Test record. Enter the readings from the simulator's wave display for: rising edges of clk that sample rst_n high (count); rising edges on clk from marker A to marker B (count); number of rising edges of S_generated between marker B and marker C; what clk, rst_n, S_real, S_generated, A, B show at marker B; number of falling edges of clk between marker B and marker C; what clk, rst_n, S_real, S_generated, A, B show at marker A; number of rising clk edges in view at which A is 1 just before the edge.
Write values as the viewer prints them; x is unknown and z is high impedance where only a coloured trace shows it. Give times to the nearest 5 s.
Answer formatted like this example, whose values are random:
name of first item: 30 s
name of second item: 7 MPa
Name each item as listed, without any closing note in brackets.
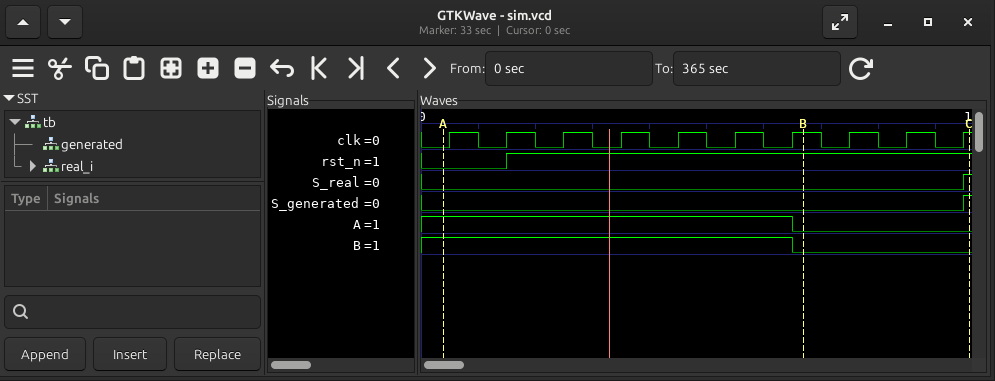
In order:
rising edges of clk that sample rst_n high: 8
rising edges on clk from marker A to marker B: 7
number of rising edges of S_generated between marker B and marker C: 1
what clk, rst_n, S_real, S_generated, A, B show at marker B: clk=1, rst_n=1, S_real=0, S_generated=0, A=0, B=0
number of falling edges of clk between marker B and marker C: 3
what clk, rst_n, S_real, S_generated, A, B show at marker A: clk=0, rst_n=0, S_real=0, S_generated=0, A=1, B=1
number of rising clk edges in view at which A is 1 just before the edge: 7
